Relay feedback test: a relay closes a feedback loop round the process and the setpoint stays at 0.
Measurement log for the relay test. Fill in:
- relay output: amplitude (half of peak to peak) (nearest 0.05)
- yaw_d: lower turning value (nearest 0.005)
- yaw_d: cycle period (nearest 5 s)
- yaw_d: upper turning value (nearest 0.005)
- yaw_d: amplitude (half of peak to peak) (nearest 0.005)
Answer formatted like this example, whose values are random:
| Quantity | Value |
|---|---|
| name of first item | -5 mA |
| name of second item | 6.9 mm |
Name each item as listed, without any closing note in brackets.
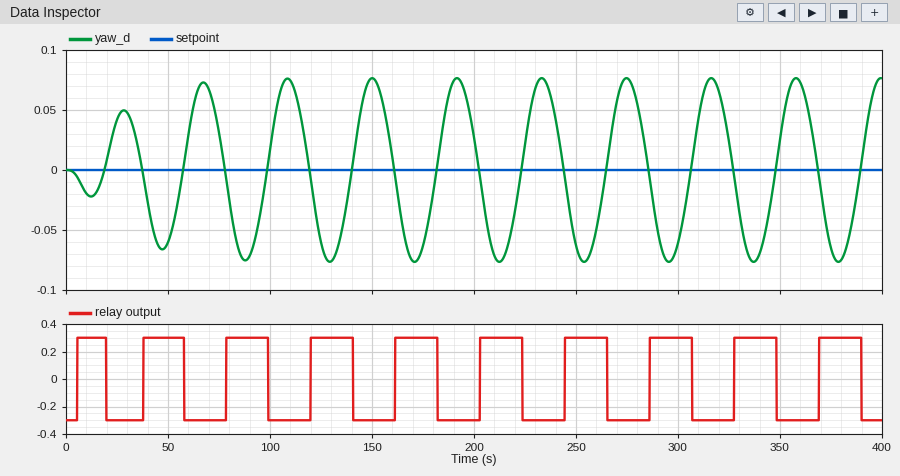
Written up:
| Quantity | Value |
|---|---|
| relay output: amplitude (half of peak to peak) | 0.30 |
| yaw_d: lower turning value | -0.075 |
| yaw_d: cycle period | 40 s |
| yaw_d: upper turning value | 0.075 |
| yaw_d: amplitude (half of peak to peak) | 0.075 |
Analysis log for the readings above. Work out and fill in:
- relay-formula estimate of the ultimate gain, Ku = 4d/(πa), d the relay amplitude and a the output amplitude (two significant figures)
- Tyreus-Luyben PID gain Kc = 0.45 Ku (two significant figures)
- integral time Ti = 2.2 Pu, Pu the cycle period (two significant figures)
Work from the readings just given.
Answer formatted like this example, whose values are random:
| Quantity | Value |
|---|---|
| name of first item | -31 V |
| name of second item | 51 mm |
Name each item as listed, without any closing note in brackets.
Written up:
| Quantity | Value |
|---|---|
| relay-formula estimate of the ultimate gain, Ku = 4d/(πa), d the relay amplitude and a the output amplitude | 5.1 |
| Tyreus-Luyben PID gain Kc = 0.45 Ku | 2.3 |
| integral time Ti = 2.2 Pu, Pu the cycle period | 88 s |
